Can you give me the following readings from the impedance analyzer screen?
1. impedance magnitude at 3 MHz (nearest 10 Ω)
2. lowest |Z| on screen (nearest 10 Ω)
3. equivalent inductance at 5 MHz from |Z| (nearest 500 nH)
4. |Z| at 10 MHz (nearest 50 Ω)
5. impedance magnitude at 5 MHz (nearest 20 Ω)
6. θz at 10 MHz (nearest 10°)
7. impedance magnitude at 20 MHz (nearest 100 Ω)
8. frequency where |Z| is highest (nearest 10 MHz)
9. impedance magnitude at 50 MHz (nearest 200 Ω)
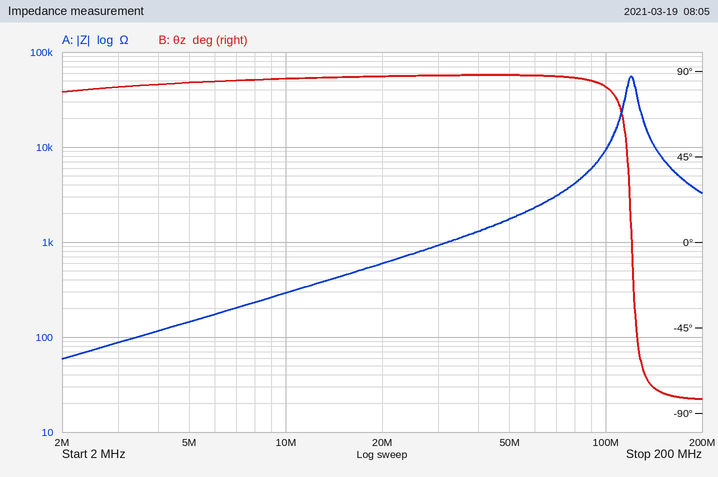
90 Ω
60 Ω
4.5 µH
300 Ω
140 Ω
90°
600 Ω
120 MHz
1.8 kΩ
